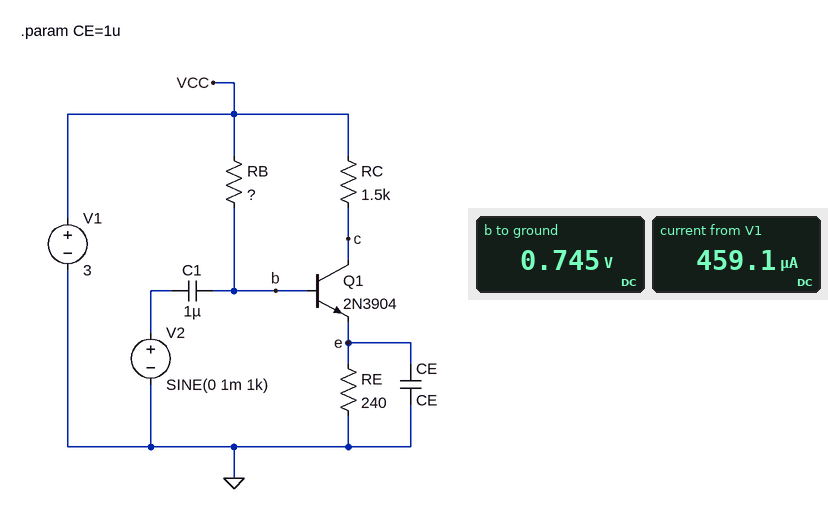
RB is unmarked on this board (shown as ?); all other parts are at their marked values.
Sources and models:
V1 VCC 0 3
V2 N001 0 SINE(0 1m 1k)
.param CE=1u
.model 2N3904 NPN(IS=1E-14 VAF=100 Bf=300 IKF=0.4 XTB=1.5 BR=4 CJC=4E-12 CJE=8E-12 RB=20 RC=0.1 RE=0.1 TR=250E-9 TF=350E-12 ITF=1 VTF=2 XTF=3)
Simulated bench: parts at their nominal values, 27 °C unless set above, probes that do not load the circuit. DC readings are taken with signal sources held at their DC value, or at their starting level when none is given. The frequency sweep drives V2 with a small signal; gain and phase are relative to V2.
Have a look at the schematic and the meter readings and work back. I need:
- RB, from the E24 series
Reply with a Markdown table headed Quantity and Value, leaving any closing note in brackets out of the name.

| Quantity | Value |
|---|---|
| RB, from the E24 series | 1.5 MΩ |
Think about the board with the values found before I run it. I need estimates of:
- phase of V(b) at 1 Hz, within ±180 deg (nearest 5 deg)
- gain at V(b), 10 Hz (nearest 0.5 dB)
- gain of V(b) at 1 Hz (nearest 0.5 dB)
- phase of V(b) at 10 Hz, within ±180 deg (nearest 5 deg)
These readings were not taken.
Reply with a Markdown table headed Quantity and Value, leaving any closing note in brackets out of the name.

| Quantity | Value |
|---|---|
| phase of V(b) at 1 Hz, within ±180 deg | 60 deg |
| gain at V(b), 10 Hz | 0 dB |
| gain of V(b) at 1 Hz | -6.5 dB |
| phase of V(b) at 10 Hz, within ±180 deg | 10 deg |
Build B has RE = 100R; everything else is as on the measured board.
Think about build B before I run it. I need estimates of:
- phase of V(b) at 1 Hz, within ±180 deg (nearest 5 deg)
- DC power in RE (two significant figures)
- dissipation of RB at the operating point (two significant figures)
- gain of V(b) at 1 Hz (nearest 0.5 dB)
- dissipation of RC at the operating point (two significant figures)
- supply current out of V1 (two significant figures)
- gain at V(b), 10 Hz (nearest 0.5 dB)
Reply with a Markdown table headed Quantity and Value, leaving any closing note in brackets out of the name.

| Quantity | Value |
|---|---|
| phase of V(b) at 1 Hz, within ±180 deg | 75 deg |
| DC power in RE | 22 µW |
| dissipation of RB at the operating point | 3.6 µW |
| gain of V(b) at 1 Hz | -11.0 dB |
| dissipation of RC at the operating point | 330 µW |
| supply current out of V1 | 470 µA |
| gain at V(b), 10 Hz | -0.5 dB |
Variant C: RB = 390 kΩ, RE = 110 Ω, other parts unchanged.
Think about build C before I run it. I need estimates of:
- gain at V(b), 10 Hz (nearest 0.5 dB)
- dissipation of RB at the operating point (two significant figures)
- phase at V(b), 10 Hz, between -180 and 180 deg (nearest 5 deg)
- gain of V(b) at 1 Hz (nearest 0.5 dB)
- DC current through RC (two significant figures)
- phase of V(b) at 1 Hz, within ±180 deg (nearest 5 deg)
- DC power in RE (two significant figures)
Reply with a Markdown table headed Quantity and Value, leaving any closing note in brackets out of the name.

| Quantity | Value |
|---|---|
| gain at V(b), 10 Hz | -1.0 dB |
| dissipation of RB at the operating point | 12 µW |
| phase at V(b), 10 Hz, between -180 and 180 deg | 25 deg |
| gain of V(b) at 1 Hz | -14.0 dB |
| DC current through RC | 1.6 mA |
| phase of V(b) at 1 Hz, within ±180 deg | 80 deg |
| DC power in RE | 300 µW |
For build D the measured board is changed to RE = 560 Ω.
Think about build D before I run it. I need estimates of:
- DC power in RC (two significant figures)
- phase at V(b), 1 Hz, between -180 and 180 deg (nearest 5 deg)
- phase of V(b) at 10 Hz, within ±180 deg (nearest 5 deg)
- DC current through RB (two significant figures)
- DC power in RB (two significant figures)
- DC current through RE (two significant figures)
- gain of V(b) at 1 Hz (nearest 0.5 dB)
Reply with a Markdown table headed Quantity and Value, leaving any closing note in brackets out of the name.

| Quantity | Value |
|---|---|
| DC power in RC | 280 µW |
| phase at V(b), 1 Hz, between -180 and 180 deg | 45 deg |
| phase of V(b) at 10 Hz, within ±180 deg | 5 deg |
| DC current through RB | 1.4 µA |
| DC power in RB | 3.0 µW |
| DC current through RE | 430 µA |
| gain of V(b) at 1 Hz | -3.0 dB |
